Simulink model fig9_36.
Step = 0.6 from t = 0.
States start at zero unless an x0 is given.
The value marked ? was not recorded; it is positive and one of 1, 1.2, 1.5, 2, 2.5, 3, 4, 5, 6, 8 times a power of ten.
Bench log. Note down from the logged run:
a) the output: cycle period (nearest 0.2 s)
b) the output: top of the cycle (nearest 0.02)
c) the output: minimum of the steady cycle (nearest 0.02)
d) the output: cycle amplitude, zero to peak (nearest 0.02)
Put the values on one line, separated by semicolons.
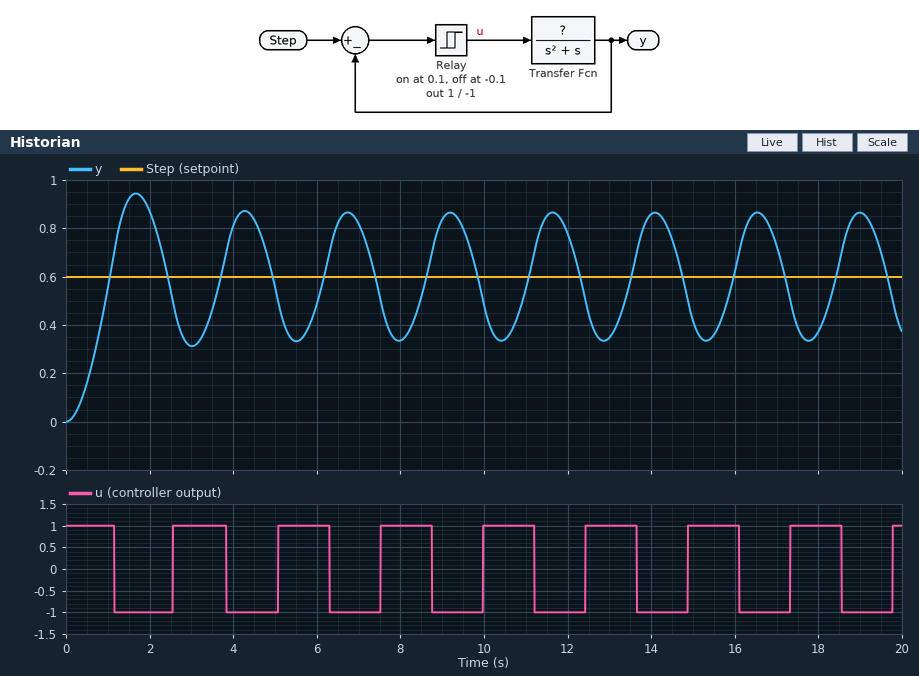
2.4 s; 0.86; 0.34; 0.26
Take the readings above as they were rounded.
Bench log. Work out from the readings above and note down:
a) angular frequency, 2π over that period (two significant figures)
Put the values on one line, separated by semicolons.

2.6 rad/s
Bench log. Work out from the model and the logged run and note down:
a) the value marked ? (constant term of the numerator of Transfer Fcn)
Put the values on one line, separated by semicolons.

1.5
